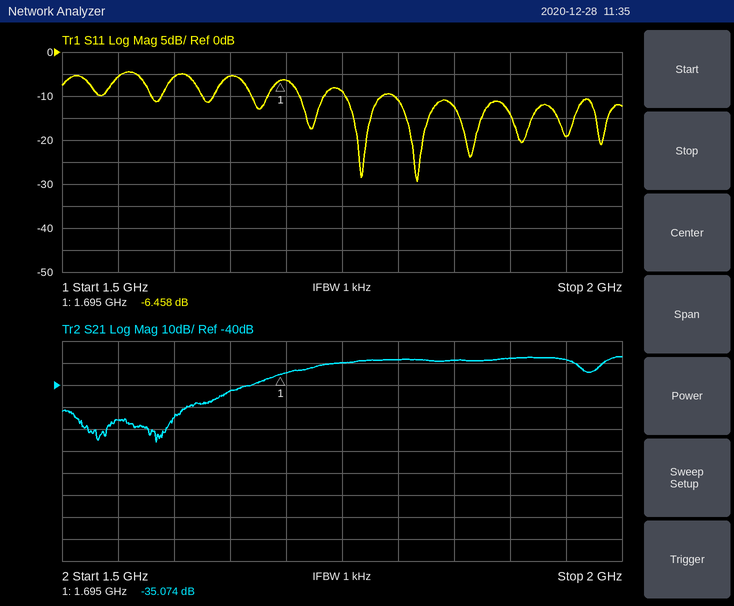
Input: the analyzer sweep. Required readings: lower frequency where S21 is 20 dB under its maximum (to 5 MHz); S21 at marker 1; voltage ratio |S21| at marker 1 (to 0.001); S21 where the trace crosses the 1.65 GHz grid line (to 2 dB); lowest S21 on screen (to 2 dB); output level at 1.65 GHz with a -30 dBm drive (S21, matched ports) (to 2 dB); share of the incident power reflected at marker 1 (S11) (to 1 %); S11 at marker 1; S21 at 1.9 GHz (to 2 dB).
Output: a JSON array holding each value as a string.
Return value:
["1.635 GHz", "-35.074 dB", "0.018", "-42 dB", "-66 dB", "-72 dBm", "23 %", "-6.458 dB", "-28 dB"]
